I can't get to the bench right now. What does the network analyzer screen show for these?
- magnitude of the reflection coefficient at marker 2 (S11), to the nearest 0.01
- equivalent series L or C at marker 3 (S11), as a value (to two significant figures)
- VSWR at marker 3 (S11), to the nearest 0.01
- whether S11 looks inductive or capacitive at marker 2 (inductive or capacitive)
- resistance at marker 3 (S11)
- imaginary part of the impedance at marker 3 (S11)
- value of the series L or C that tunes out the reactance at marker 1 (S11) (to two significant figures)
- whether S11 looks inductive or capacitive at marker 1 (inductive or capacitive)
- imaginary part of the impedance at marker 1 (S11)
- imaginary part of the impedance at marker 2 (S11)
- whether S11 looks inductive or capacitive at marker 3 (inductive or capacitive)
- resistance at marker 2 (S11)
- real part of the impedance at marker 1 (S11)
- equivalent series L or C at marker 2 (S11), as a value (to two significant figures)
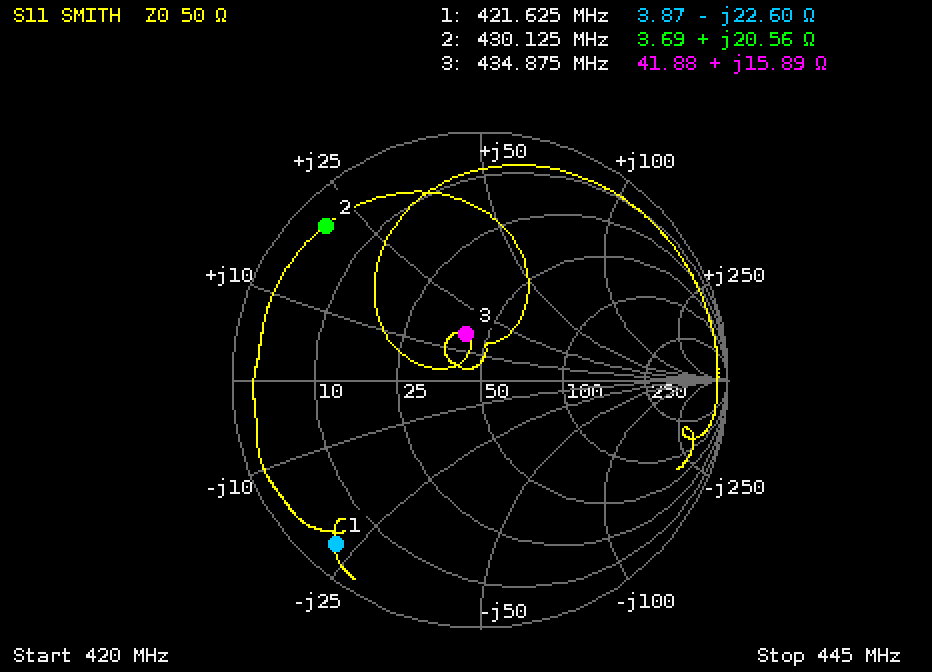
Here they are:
0.88
5.8 nH
1.47
inductive
41.88 Ω
+15.89 Ω
8.5 nH
capacitive
-22.60 Ω
+20.56 Ω
inductive
3.69 Ω
3.87 Ω
7.6 nH
